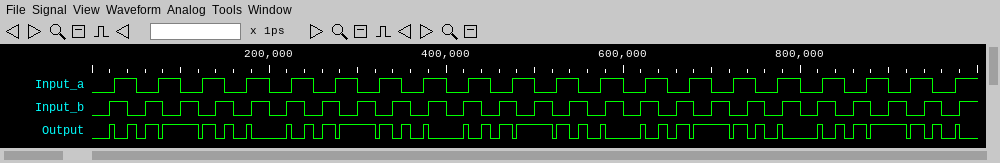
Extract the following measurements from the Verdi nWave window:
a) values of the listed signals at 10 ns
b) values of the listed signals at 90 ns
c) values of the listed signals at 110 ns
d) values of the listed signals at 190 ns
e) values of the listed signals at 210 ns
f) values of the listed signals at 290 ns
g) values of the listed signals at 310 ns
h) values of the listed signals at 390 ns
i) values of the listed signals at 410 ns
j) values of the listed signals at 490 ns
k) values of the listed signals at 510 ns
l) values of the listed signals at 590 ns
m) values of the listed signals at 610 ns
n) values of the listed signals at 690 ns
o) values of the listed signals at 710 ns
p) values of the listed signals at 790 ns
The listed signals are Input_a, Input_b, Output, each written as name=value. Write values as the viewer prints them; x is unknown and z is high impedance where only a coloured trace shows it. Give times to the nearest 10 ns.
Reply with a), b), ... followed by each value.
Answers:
a) Input_a=0, Input_b=0, Output=0
b) Input_a=1, Input_b=0, Output=1
c) Input_a=0, Input_b=1, Output=1
d) Input_a=1, Input_b=1, Output=0
e) Input_a=0, Input_b=0, Output=0
f) Input_a=1, Input_b=0, Output=1
g) Input_a=0, Input_b=1, Output=1
h) Input_a=1, Input_b=1, Output=0
i) Input_a=0, Input_b=0, Output=0
j) Input_a=1, Input_b=0, Output=1
k) Input_a=0, Input_b=1, Output=1
l) Input_a=1, Input_b=1, Output=0
m) Input_a=0, Input_b=0, Output=0
n) Input_a=1, Input_b=0, Output=1
o) Input_a=0, Input_b=1, Output=1
p) Input_a=1, Input_b=1, Output=0
